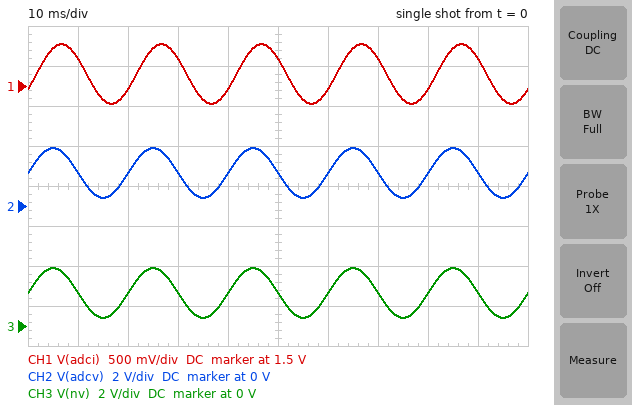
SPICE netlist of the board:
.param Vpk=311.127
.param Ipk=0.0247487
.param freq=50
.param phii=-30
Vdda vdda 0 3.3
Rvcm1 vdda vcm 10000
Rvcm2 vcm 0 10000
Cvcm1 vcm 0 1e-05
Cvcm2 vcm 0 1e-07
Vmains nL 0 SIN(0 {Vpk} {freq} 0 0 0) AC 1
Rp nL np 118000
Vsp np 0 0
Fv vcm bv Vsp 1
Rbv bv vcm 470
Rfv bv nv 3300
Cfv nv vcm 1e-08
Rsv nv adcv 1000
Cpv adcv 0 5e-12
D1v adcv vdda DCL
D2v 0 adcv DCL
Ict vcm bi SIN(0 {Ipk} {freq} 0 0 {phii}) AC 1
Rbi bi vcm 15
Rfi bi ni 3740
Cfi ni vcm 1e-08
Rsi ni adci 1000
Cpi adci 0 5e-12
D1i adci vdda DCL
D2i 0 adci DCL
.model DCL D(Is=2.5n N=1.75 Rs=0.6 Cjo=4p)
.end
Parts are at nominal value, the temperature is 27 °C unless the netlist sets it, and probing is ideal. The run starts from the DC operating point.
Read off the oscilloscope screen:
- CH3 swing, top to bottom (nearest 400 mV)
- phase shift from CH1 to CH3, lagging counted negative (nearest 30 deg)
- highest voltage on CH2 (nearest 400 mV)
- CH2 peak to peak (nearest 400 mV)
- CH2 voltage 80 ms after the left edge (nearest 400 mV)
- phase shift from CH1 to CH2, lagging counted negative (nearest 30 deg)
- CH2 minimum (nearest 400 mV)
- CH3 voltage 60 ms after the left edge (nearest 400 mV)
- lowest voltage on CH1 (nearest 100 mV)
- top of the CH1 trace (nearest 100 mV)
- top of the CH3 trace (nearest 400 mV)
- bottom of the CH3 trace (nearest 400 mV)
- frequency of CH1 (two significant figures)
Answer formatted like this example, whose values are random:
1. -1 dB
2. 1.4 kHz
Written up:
1. 2.4 V
2. 30 deg
3. 2.8 V
4. 2.4 V
5. 1.6 V
6. 30 deg
7. 400 mV
8. 1.6 V
9. 1.3 V
10. 2.0 V
11. 2.8 V
12. 400 mV
13. 50 Hz
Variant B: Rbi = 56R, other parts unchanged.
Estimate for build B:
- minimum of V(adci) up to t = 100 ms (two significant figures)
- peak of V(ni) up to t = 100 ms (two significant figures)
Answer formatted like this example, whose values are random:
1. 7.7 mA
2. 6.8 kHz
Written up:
1. 260 mV
2. 3.0 V
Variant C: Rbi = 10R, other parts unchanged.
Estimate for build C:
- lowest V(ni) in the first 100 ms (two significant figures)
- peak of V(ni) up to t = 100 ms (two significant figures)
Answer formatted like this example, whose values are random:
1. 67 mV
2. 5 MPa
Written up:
1. 1.4 V
2. 1.9 V
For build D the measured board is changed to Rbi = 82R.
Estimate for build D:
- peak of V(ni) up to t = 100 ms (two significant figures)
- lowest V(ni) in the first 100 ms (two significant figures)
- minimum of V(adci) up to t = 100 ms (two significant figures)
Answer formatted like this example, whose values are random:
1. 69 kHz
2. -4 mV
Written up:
1. 3.7 V
2. -360 mV
3. -350 mV
